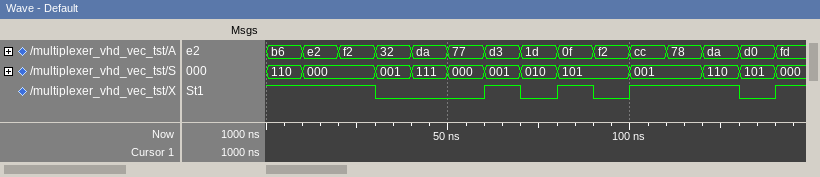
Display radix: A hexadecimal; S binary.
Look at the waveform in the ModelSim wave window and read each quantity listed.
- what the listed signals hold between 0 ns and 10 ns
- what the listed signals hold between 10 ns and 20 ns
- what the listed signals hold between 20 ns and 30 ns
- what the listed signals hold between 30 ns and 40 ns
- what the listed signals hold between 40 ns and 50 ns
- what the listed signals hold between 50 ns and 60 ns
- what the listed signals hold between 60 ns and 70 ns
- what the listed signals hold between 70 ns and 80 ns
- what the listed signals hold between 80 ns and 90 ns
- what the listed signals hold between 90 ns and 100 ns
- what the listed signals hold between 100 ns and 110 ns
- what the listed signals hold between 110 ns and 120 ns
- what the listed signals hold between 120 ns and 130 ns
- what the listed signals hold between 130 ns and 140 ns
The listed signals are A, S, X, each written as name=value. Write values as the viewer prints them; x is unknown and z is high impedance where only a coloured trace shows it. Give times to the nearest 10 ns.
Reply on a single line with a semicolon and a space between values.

A=b6, S=110, X=1; A=e2, S=000, X=1; A=f2, S=000, X=1; A=32, S=001, X=0; A=da, S=111, X=0; A=77, S=000, X=0; A=d3, S=001, X=1; A=1d, S=010, X=0; A=0f, S=101, X=1; A=f2, S=101, X=0; A=cc, S=001, X=1; A=78, S=001, X=1; A=da, S=110, X=1; A=d0, S=101, X=0
